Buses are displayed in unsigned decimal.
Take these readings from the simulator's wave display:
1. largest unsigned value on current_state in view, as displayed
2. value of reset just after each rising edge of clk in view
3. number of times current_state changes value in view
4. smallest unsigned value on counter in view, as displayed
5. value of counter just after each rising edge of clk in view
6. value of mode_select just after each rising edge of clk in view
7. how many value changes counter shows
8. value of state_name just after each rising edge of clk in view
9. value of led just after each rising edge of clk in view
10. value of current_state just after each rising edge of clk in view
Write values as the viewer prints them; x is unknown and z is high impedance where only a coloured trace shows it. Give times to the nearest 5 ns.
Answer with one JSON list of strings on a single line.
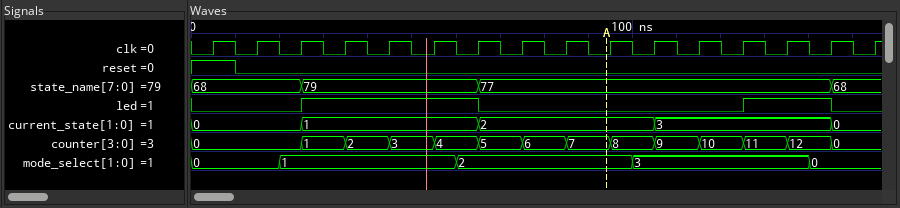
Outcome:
["3", "1 0 0 0 0 0 0 0 0 0 0 0 0 0 0 0", "4", "0", "0, 0, 1, 2, 3, 4, 5, 6, 7, 8, 9, 10, 11, 12, 0, 0", "0, 0, 1, 1, 1, 1, 2, 2, 2, 2, 3, 3, 3, 3, 0, 0", "13", "68, 68, 79, 79, 79, 79, 77, 77, 77, 77, 77, 77, 77, 77, 68, 68", "0 0 1 1 1 1 0 0 0 0 0 0 1 1 0 0", "0, 0, 1, 1, 1, 1, 2, 2, 2, 2, 3, 3, 3, 3, 0, 0"]
